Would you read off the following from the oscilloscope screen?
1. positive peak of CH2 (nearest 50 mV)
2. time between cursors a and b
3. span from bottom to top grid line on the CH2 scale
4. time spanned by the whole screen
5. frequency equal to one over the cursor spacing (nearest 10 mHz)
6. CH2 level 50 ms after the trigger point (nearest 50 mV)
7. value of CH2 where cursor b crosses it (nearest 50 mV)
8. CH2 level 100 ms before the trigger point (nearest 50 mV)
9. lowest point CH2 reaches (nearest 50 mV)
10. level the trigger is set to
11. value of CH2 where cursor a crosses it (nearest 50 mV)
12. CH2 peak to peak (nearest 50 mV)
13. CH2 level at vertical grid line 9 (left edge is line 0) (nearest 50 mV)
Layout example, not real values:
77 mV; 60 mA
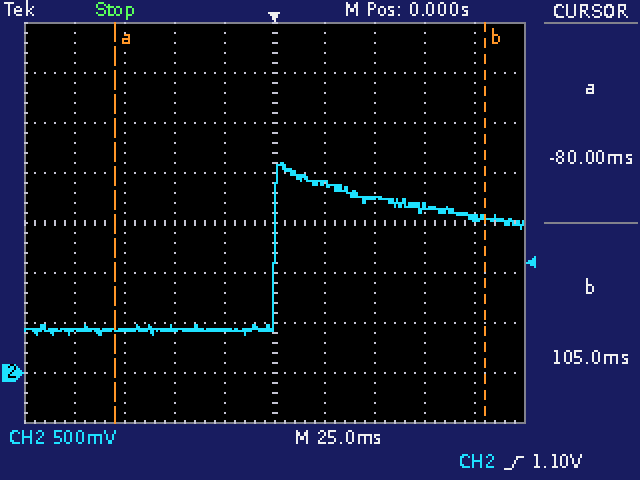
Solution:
2.10 V; 185.0 ms; 4 V; 250 ms; 5.41 Hz; 1.75 V; 1.55 V; 450 mV; 400 mV; 1.10 V; 450 mV; 1.70 V; 1.55 V
